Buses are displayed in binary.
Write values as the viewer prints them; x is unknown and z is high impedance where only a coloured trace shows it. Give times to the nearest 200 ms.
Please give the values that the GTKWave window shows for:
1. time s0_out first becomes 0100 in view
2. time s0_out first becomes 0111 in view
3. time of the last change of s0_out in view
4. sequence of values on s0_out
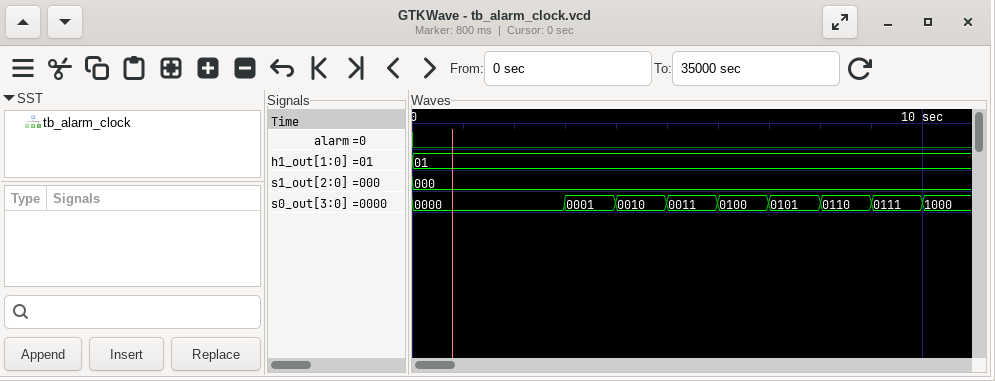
6000 ms
9000 ms
10000 ms
0000, 0001, 0010, 0011, 0100, 0101, 0110, 0111, 1000
